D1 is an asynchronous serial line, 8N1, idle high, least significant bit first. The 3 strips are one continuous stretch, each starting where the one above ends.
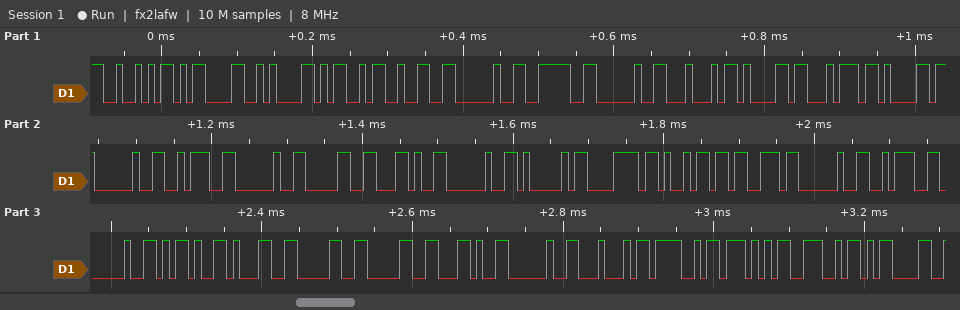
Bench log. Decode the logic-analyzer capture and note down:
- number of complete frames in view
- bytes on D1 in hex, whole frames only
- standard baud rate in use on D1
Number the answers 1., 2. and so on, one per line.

1. 36
2. 52 0D 0A 4D 32 20 3E 20 44 61 74 61 20 3A 20 30 2C 20 41 78 69 73 20 3A 20 2D 31 30 30 2C 20 44 4F 57 4E 0D
3. 115200 baud
